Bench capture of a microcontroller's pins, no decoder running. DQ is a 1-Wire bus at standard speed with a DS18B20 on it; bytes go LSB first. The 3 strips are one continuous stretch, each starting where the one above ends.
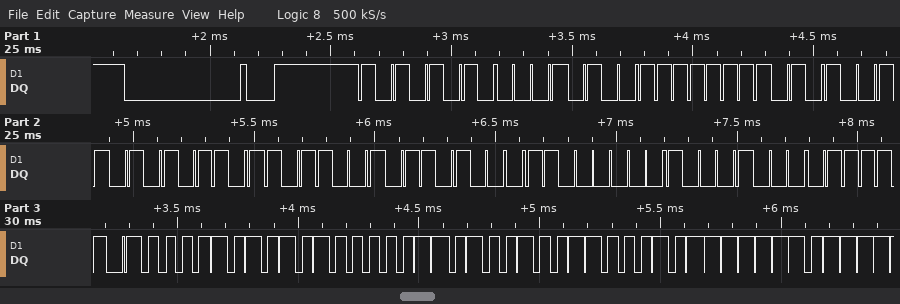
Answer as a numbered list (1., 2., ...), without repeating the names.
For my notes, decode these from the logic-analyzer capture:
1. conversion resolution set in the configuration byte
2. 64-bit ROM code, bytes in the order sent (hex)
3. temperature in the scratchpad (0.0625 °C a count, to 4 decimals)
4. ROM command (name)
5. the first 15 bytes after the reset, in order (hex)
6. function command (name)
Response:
1. 12 bits
2. 28 FF CA 6A 9B 16 03 11
3. 85.0000 °C
4. Match ROM
5. 55 28 FF CA 6A 9B 16 03 11 BE 50 05 4B 46 7F
6. Read Scratchpad
